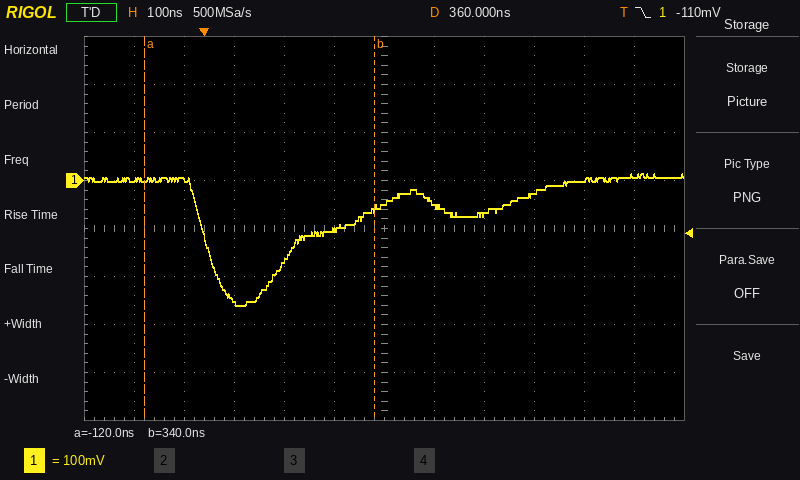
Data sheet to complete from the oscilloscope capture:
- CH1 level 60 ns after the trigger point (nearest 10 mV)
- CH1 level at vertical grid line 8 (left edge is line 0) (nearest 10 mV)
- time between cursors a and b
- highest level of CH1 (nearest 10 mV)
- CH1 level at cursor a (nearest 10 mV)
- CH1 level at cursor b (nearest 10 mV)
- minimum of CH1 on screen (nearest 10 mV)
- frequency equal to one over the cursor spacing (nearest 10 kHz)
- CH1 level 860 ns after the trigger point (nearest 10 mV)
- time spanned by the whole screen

-250 mV
-70 mV
460 ns
10 mV
0 mV
-60 mV
-260 mV
2.17 MHz
10 mV
1.2 µs
